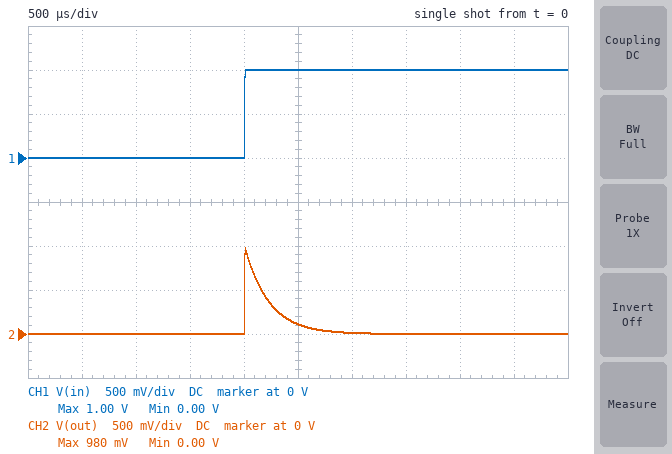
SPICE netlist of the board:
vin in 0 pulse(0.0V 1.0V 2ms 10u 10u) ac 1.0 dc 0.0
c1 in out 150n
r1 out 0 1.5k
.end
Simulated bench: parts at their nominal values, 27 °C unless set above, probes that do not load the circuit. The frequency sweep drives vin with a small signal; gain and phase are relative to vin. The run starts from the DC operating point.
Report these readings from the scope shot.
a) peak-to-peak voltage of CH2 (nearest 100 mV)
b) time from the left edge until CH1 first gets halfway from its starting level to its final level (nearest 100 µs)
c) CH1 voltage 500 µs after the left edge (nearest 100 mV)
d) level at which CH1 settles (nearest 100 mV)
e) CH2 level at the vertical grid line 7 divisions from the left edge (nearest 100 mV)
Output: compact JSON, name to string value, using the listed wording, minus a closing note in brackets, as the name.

{"peak-to-peak voltage of CH2": "1.0 V", "time from the left edge until CH1 first gets halfway from its starting level to its final level": "2.0 ms", "CH1 voltage 500 µs after the left edge": "0 V", "level at which CH1 settles": "1.0 V", "CH2 level at the vertical grid line 7 divisions from the left edge": "0 V"}
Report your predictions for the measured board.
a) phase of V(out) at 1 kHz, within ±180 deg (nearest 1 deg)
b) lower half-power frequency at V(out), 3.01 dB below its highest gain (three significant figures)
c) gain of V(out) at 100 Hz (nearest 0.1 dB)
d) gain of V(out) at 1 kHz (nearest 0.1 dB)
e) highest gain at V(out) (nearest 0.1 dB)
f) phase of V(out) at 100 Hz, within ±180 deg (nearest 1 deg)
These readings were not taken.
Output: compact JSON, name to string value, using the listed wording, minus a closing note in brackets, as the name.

{"phase of V(out) at 1 kHz, within ±180 deg": "35 deg", "lower half-power frequency at V(out), 3.01 dB below its highest gain": "707 Hz", "gain of V(out) at 100 Hz": "-17.1 dB", "gain of V(out) at 1 kHz": "-1.8 dB", "highest gain at V(out)": "0 dB", "phase of V(out) at 100 Hz, within ±180 deg": "82 deg"}
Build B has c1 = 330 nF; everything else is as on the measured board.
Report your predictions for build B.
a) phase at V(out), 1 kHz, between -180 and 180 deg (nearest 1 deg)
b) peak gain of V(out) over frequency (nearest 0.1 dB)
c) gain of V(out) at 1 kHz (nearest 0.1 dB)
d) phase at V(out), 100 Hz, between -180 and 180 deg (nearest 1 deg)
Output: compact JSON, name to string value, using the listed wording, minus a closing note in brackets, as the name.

{"phase at V(out), 1 kHz, between -180 and 180 deg": "18 deg", "peak gain of V(out) over frequency": "0 dB", "gain of V(out) at 1 kHz": "-0.4 dB", "phase at V(out), 100 Hz, between -180 and 180 deg": "73 deg"}
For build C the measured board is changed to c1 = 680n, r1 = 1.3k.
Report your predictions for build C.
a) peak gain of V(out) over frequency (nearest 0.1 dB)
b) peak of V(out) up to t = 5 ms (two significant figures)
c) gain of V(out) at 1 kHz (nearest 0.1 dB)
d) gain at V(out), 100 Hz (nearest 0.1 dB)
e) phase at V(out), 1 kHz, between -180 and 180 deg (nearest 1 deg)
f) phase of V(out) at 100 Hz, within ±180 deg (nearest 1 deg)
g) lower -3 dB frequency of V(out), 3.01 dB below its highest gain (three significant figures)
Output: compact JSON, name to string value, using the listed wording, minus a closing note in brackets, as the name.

{"peak gain of V(out) over frequency": "0 dB", "peak of V(out) up to t = 5 ms": "990 mV", "gain of V(out) at 1 kHz": "-0.1 dB", "gain at V(out), 100 Hz": "-6.3 dB", "phase at V(out), 1 kHz, between -180 and 180 deg": "10 deg", "phase of V(out) at 100 Hz, within ±180 deg": "61 deg", "lower -3 dB frequency of V(out), 3.01 dB below its highest gain": "180 Hz"}
